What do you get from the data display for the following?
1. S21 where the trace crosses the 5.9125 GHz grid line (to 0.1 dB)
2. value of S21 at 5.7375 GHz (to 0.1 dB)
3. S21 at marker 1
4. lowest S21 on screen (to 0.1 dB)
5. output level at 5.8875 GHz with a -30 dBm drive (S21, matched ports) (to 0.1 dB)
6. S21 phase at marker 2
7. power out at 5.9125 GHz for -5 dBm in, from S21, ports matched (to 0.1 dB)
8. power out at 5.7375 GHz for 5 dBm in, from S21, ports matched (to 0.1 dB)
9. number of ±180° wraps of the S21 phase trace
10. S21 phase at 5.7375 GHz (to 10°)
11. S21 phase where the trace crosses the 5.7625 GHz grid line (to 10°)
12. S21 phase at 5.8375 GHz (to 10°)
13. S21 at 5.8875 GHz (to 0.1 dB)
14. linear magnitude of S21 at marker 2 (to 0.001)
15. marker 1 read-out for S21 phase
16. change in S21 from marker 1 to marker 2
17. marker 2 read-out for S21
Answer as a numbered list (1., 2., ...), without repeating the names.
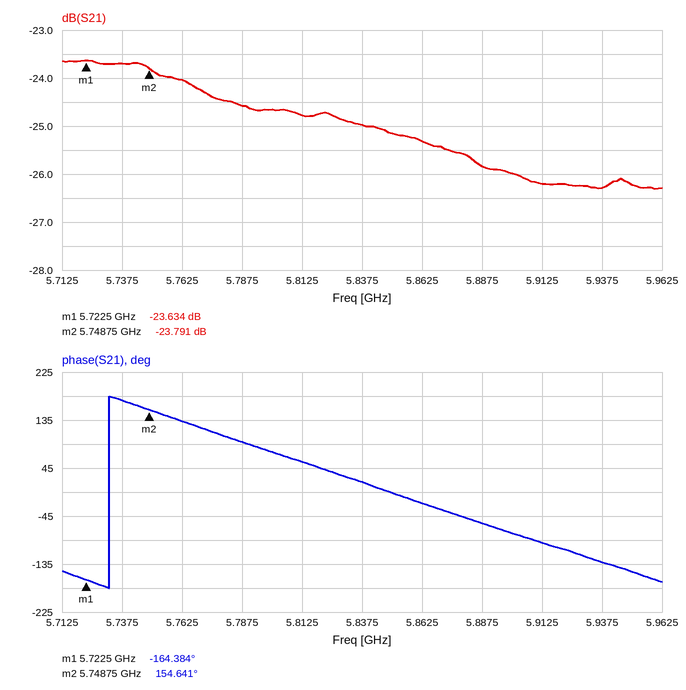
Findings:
1. -26.2 dB
2. -23.7 dB
3. -23.634 dB
4. -26.3 dB
5. -55.8 dBm
6. 154.641°
7. -31.2 dBm
8. -18.7 dBm
9. 1
10. 170°
11. 130°
12. 20°
13. -25.8 dB
14. 0.065
15. -164.384°
16. -0.157 dB
17. -23.791 dB
